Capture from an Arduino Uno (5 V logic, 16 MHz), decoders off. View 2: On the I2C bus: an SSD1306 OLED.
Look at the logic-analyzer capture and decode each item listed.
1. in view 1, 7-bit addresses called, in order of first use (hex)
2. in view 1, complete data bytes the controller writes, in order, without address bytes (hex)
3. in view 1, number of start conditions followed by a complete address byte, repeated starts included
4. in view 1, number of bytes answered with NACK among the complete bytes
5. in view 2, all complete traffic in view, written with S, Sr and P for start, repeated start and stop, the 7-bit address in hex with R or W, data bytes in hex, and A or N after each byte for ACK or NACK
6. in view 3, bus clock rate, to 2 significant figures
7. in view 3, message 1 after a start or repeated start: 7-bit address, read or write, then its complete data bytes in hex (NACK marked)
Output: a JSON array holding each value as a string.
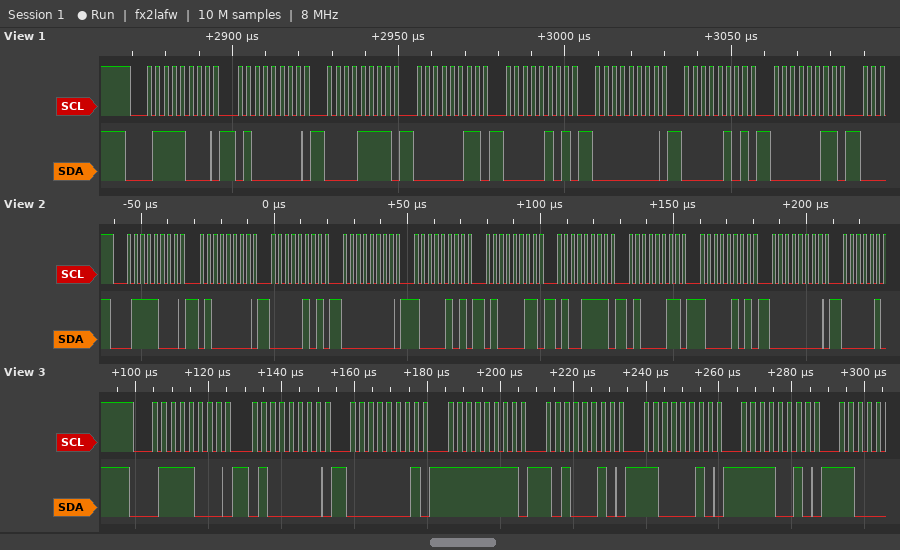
["0x3C", "40 0F 03 05 00 05 03", "1", "0", "S 3CW A 40 A 05 A 00 A 85 A 43 A 4F A 43 A 85 A 00 A", "400 kHz", "0x3C write: 40 01 FF A2 C2 F2"]
